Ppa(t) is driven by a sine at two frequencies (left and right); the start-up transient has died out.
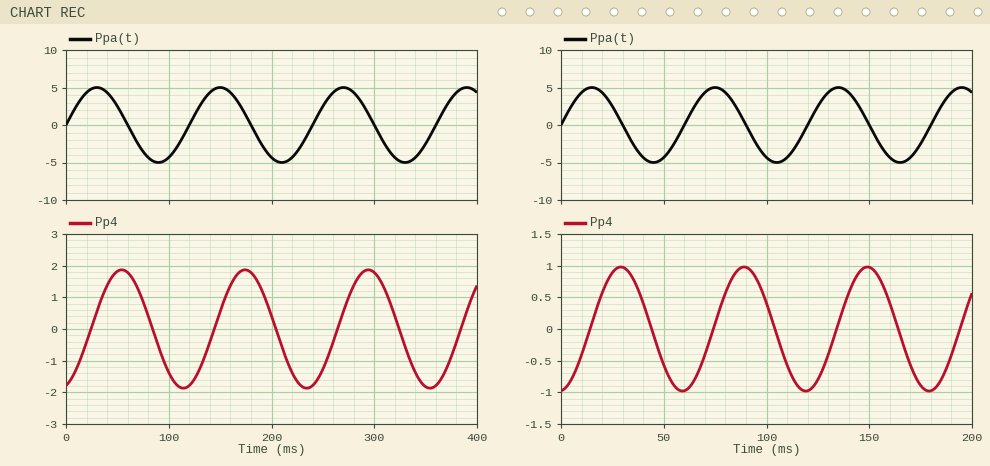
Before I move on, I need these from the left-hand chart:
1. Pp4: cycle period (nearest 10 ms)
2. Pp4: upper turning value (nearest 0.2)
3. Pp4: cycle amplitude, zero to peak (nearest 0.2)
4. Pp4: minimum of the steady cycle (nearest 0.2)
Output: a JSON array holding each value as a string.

["120 ms", "1.8", "1.8", "-1.8"]
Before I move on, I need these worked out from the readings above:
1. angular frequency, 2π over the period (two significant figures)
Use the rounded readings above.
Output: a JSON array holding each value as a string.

["0.052 rad/ms"]
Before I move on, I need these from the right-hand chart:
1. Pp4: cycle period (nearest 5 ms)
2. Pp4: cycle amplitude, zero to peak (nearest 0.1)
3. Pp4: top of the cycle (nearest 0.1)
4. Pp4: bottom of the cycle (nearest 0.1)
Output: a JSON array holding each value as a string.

["60 ms", "1.0", "1.0", "-1.0"]
